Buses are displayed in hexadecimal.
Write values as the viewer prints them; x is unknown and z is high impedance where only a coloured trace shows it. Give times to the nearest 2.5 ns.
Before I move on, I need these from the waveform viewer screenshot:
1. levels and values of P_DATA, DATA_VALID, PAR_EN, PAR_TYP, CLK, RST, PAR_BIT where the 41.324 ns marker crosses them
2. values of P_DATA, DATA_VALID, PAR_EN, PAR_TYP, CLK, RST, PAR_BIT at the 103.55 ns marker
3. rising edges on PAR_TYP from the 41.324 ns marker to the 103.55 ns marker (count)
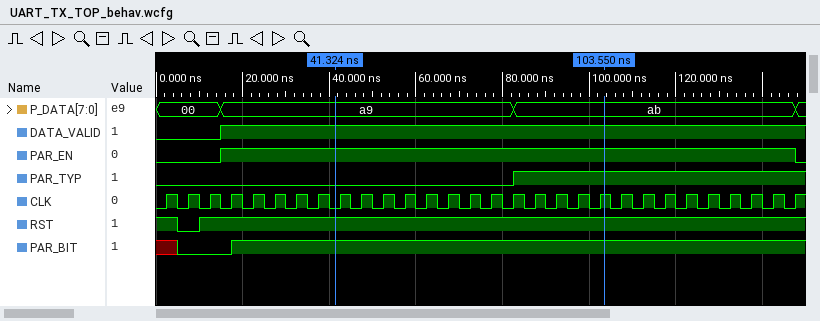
P_DATA=a9, DATA_VALID=1, PAR_EN=1, PAR_TYP=0, CLK=0, RST=1, PAR_BIT=1
P_DATA=ab, DATA_VALID=1, PAR_EN=1, PAR_TYP=1, CLK=1, RST=1, PAR_BIT=1
1
